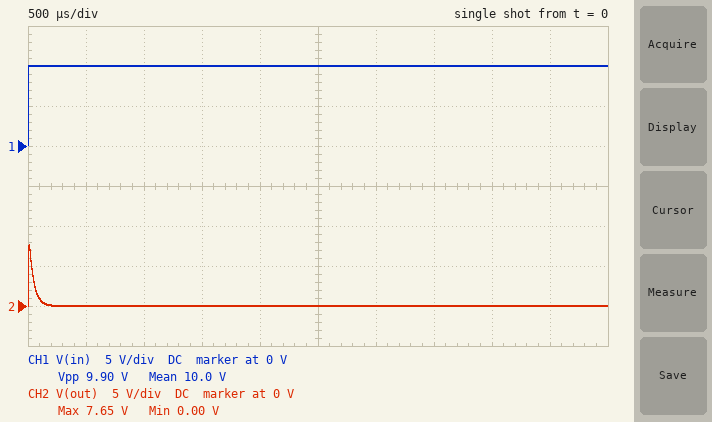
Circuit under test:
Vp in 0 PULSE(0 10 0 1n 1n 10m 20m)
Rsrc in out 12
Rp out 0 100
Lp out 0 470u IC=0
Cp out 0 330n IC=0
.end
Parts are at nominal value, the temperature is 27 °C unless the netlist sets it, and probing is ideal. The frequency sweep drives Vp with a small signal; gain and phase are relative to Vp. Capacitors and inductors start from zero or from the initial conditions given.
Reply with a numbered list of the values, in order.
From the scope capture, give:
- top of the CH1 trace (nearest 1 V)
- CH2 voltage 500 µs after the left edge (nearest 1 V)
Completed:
1. 10 V
2. 0 V
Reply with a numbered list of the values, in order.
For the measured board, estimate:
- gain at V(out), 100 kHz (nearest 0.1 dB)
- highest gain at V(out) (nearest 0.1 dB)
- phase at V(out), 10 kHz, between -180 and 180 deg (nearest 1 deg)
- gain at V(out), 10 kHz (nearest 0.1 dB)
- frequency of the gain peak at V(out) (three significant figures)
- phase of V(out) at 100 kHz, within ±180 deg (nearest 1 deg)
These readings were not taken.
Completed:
1. -8.6 dB
2. -1.0 dB
3. 8 deg
4. -1.1 dB
5. 12.8 kHz
6. -65 deg
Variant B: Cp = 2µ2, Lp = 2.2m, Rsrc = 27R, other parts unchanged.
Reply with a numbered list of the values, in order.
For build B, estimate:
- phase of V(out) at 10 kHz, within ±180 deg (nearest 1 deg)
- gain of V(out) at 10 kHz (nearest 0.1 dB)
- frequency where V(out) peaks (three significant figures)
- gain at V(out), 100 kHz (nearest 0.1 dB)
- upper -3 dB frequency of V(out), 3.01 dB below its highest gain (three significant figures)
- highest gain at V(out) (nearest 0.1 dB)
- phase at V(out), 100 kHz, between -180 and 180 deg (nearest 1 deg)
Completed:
1. -70 deg
2. -11.5 dB
3. 2.29 kHz
4. -31.4 dB
5. 4.55 kHz
6. -2.1 dB
7. -88 deg
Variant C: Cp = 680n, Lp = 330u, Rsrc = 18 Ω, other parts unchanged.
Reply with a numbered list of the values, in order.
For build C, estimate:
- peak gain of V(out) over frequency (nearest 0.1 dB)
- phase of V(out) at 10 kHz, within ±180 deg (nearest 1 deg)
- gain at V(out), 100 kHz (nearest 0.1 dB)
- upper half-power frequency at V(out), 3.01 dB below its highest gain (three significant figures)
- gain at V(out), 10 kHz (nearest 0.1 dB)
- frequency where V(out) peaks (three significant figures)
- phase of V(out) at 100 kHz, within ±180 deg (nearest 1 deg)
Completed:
1. -1.4 dB
2. 5 deg
3. -17.7 dB
4. 20.8 kHz
5. -1.5 dB
6. 10.6 kHz
7. -81 deg
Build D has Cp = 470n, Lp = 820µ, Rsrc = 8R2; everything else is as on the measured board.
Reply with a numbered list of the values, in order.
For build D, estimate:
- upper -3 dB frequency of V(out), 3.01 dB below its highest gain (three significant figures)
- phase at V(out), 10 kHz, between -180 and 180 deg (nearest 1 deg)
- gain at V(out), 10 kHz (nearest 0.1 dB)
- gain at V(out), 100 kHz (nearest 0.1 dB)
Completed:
1. 46.1 kHz
2. -4 deg
3. -0.7 dB
4. -8.4 dB
